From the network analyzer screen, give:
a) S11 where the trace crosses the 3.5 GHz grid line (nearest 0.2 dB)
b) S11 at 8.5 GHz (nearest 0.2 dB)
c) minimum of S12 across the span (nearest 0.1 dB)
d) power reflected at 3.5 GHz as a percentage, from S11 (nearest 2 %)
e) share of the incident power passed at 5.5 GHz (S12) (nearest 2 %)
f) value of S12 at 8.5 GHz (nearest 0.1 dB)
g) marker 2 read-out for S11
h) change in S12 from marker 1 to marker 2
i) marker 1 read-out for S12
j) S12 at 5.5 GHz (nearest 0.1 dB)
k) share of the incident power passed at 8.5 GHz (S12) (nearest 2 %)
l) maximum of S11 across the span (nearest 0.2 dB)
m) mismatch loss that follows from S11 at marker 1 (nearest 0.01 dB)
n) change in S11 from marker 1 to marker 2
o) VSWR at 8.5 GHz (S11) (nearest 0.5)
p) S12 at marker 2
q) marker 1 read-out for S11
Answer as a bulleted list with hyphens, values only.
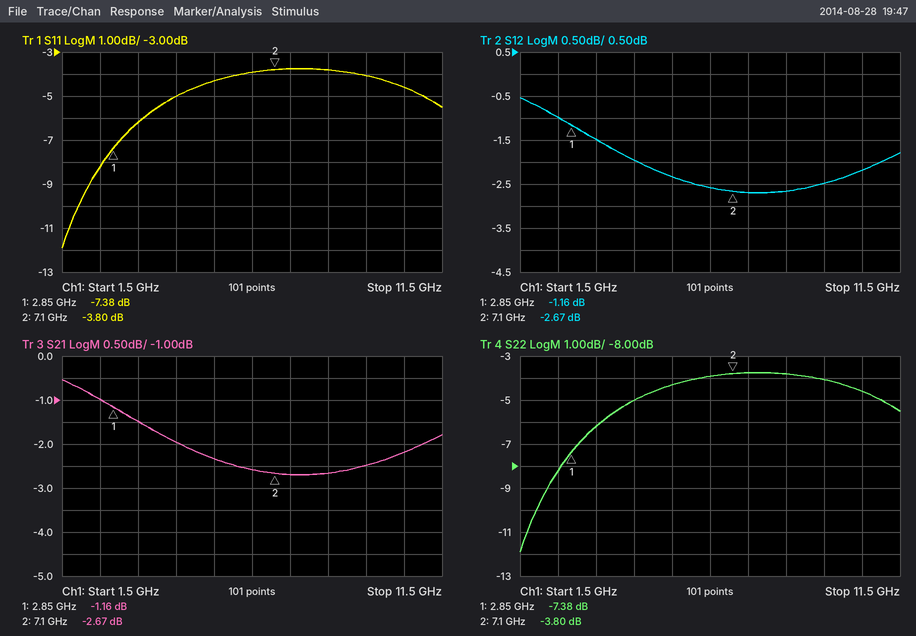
- -6.2 dB
- -3.8 dB
- -2.7 dB
- 24 %
- 58 %
- -2.7 dB
- -3.80 dB
- -1.51 dB
- -1.16 dB
- -2.3 dB
- 54 %
- -3.8 dB
- 0.88 dB
- 3.58 dB
- 4.5
- -2.67 dB
- -7.38 dB
